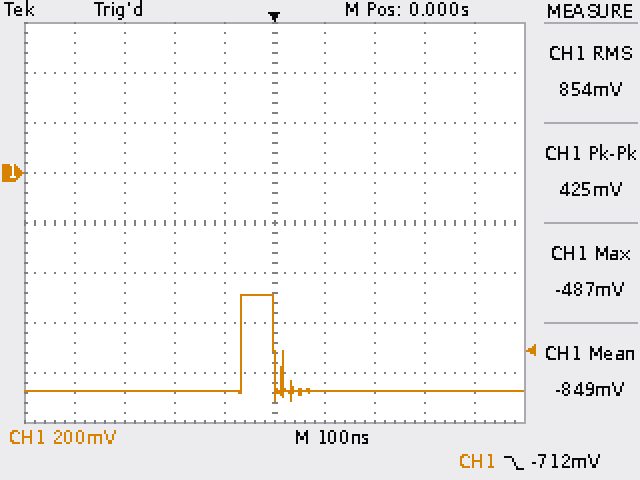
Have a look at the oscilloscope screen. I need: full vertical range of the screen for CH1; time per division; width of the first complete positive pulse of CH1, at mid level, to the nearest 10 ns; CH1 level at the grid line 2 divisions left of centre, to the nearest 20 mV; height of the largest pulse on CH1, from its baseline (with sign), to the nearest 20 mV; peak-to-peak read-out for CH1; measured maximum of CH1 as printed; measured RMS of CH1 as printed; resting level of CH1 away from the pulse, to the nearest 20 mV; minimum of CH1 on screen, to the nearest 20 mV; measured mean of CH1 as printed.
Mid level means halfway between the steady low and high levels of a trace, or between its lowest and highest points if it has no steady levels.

1.6 V
100 ns
70 ns
-880 mV
+380 mV
425 mV
-487 mV
854 mV
-880 mV
-920 mV
-849 mV
